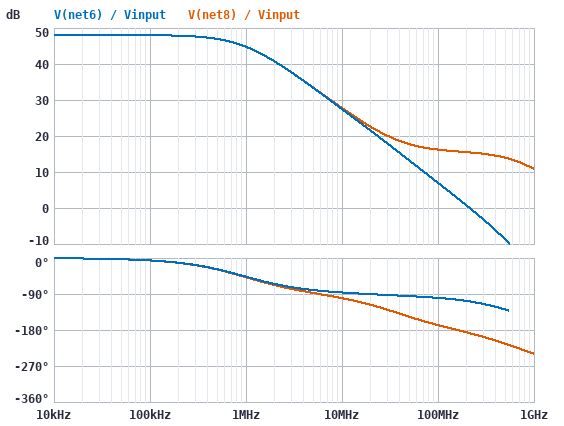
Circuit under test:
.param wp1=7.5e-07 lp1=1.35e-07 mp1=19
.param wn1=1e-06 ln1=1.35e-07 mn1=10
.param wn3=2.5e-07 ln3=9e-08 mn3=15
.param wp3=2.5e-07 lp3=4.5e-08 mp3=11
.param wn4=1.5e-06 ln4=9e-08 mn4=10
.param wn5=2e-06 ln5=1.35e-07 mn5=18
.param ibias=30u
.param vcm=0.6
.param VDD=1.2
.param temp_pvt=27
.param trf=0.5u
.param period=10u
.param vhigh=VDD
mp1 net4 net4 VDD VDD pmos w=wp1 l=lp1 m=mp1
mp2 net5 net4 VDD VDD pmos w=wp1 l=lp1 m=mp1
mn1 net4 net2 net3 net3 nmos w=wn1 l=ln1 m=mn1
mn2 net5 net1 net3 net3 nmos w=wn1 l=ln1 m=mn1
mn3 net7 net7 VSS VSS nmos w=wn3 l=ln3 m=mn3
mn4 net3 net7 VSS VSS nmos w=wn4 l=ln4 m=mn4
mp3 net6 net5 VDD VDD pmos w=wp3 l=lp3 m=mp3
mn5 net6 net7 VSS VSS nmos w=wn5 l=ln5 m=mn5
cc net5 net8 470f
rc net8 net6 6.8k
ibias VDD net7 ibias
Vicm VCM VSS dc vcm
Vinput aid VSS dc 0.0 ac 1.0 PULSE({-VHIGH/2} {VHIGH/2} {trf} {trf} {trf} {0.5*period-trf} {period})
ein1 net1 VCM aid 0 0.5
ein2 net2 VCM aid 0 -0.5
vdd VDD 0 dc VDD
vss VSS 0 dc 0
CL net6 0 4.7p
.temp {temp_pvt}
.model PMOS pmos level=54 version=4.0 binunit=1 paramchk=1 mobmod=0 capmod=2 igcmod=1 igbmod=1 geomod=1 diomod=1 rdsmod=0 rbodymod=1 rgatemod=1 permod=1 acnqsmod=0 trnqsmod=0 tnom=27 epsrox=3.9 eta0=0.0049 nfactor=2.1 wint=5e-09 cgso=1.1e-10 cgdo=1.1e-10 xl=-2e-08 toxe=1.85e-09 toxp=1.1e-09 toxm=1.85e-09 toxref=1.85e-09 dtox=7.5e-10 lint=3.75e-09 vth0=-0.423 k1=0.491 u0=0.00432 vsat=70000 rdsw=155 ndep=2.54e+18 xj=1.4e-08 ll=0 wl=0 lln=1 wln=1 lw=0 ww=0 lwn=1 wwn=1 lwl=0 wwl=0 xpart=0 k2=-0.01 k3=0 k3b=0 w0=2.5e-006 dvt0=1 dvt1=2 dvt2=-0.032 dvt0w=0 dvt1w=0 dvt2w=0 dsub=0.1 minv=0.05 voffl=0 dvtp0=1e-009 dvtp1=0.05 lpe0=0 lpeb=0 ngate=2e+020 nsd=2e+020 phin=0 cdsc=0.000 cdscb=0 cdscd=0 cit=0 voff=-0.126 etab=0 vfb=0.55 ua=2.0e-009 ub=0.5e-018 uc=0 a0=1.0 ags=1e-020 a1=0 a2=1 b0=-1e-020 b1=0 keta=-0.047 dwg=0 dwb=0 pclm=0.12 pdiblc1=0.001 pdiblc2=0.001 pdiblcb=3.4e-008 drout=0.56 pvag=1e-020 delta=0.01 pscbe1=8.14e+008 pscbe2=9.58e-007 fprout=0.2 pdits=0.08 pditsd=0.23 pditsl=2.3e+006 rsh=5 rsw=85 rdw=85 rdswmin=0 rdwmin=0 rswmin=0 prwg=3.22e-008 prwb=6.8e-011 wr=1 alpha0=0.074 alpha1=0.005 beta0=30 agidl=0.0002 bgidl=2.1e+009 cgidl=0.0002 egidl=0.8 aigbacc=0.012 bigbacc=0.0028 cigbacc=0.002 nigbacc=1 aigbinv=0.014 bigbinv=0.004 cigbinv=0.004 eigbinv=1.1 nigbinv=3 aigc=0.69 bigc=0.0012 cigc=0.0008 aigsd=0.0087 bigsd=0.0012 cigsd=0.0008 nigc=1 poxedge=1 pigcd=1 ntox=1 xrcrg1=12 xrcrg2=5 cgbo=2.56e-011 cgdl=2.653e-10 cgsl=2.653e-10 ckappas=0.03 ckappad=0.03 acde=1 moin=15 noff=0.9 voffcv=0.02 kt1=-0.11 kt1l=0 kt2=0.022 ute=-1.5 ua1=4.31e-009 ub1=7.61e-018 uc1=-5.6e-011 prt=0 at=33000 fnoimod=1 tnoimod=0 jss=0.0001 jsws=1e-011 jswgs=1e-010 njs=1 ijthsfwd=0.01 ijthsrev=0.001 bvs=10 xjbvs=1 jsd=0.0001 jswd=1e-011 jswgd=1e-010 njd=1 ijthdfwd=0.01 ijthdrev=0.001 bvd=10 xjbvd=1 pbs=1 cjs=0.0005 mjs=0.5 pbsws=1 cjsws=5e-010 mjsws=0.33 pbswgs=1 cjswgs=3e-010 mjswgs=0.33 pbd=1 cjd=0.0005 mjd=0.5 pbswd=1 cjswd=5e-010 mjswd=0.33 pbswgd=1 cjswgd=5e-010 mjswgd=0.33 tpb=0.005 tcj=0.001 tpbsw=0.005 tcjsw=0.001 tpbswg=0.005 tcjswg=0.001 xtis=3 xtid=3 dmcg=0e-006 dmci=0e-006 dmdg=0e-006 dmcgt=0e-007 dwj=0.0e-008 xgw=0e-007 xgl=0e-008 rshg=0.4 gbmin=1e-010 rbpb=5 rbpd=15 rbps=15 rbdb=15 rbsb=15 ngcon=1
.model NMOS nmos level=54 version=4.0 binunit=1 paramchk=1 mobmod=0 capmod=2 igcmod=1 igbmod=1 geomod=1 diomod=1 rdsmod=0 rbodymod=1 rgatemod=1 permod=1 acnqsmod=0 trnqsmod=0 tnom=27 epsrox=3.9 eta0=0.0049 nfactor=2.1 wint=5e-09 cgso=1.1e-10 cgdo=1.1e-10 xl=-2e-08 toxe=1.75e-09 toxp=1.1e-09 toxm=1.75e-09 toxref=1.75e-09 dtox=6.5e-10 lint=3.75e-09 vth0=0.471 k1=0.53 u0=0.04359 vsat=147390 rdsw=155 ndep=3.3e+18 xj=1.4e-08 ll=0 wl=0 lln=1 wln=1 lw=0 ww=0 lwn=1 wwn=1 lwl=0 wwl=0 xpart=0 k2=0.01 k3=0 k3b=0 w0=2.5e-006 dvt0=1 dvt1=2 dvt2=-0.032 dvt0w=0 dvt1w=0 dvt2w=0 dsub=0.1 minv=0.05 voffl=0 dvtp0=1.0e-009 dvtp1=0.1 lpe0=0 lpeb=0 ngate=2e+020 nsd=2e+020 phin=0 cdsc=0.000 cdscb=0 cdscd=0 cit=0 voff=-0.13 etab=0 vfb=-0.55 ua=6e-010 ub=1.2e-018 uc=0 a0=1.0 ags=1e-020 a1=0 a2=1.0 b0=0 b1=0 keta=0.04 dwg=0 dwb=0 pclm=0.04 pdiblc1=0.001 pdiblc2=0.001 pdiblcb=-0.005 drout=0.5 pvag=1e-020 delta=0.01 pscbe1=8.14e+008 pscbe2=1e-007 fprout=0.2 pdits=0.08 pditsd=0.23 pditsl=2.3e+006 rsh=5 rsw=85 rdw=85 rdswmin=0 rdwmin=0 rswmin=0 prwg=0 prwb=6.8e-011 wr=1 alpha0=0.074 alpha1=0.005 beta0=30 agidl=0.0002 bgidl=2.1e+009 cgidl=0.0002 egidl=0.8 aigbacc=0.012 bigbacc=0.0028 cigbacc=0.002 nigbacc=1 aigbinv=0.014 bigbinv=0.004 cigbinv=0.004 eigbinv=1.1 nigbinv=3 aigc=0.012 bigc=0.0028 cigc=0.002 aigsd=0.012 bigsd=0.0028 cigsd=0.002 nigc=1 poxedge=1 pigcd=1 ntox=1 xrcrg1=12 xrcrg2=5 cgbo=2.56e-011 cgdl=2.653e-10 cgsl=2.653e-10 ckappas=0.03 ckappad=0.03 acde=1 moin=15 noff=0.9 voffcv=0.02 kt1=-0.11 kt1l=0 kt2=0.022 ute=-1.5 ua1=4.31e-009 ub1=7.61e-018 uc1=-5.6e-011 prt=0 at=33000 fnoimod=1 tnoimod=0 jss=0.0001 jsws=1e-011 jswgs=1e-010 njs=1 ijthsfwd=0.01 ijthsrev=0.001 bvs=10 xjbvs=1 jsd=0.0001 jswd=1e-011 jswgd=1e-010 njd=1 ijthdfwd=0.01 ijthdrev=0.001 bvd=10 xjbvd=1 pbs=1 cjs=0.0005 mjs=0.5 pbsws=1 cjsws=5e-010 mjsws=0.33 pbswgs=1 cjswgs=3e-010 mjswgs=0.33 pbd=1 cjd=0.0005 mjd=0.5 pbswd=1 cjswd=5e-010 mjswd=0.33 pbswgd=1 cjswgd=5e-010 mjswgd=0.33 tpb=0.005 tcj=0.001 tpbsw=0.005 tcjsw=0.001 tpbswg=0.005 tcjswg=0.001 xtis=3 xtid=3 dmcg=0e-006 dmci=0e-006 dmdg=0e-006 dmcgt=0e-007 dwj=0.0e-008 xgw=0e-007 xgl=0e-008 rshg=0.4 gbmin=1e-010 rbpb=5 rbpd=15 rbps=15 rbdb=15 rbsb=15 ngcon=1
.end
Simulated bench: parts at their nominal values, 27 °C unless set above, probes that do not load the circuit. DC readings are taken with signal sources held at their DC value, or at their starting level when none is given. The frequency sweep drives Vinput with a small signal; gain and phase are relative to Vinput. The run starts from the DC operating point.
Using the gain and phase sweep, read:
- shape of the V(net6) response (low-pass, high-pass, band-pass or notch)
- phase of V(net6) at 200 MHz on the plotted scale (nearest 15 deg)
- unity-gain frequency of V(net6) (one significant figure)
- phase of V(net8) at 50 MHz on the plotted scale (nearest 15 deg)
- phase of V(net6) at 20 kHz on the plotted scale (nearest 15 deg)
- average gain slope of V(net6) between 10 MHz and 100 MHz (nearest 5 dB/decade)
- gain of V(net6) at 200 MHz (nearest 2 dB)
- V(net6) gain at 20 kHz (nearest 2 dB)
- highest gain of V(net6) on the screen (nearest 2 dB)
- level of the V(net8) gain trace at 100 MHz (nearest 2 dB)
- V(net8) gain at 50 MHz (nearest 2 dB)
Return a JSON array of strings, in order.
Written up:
["low-pass", "-105 deg", "200 MHz", "-150 deg", "0 deg", "-20 dB/decade", "0 dB", "48 dB", "48 dB", "16 dB", "18 dB"]
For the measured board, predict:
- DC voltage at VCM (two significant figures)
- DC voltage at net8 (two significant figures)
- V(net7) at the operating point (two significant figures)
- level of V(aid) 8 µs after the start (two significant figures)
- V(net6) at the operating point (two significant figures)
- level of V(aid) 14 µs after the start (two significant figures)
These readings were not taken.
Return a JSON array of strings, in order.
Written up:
["600 mV", "730 mV", "440 mV", "-600 mV", "730 mV", "600 mV"]
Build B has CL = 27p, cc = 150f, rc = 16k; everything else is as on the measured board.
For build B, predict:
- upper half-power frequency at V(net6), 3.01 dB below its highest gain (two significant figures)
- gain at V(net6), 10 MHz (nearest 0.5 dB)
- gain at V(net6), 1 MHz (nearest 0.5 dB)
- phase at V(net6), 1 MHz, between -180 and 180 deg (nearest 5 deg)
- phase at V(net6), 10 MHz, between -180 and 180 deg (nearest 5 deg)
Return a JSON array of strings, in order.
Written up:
["1.3 MHz", "29.0 dB", "46.0 dB", "-40 deg", "-105 deg"]
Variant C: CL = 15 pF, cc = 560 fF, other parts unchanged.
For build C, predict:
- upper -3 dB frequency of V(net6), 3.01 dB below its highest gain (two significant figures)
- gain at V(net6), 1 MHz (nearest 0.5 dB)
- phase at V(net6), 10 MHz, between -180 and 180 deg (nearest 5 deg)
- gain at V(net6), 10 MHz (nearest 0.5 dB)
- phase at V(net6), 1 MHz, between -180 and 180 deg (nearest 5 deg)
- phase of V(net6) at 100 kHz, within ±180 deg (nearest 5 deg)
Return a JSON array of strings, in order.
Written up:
["710 kHz", "43.5 dB", "-105 deg", "24.0 dB", "-55 deg", "-10 deg"]
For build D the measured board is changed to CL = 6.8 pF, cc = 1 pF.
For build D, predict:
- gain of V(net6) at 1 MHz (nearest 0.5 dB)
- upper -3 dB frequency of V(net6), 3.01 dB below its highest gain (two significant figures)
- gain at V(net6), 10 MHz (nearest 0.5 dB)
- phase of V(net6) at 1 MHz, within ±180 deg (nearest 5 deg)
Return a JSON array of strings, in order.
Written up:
["40.5 dB", "460 kHz", "21.5 dB", "-65 deg"]
